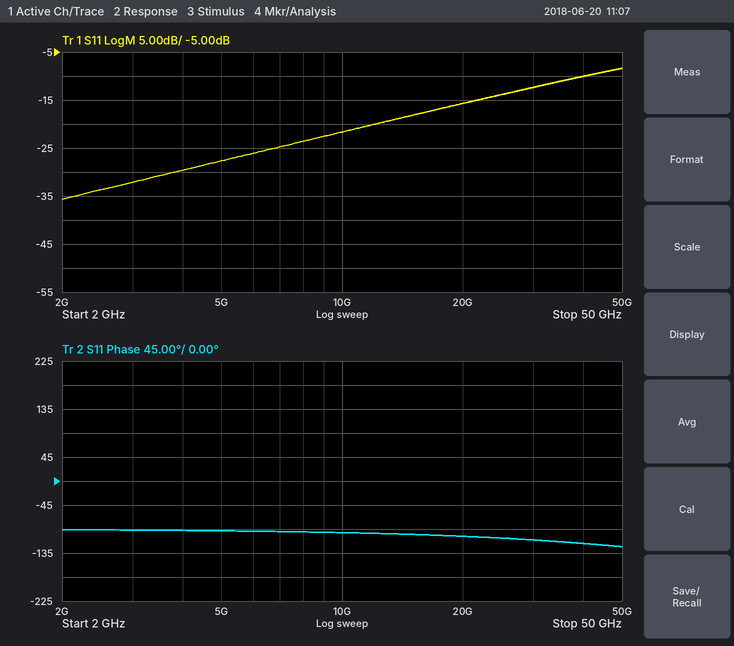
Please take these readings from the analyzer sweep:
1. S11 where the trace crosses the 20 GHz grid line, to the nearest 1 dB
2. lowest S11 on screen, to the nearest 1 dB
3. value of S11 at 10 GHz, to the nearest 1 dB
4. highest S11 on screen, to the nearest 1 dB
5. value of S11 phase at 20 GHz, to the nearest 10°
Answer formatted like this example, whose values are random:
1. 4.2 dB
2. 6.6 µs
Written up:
1. -16 dB
2. -36 dB
3. -22 dB
4. -8 dB
5. -100°
